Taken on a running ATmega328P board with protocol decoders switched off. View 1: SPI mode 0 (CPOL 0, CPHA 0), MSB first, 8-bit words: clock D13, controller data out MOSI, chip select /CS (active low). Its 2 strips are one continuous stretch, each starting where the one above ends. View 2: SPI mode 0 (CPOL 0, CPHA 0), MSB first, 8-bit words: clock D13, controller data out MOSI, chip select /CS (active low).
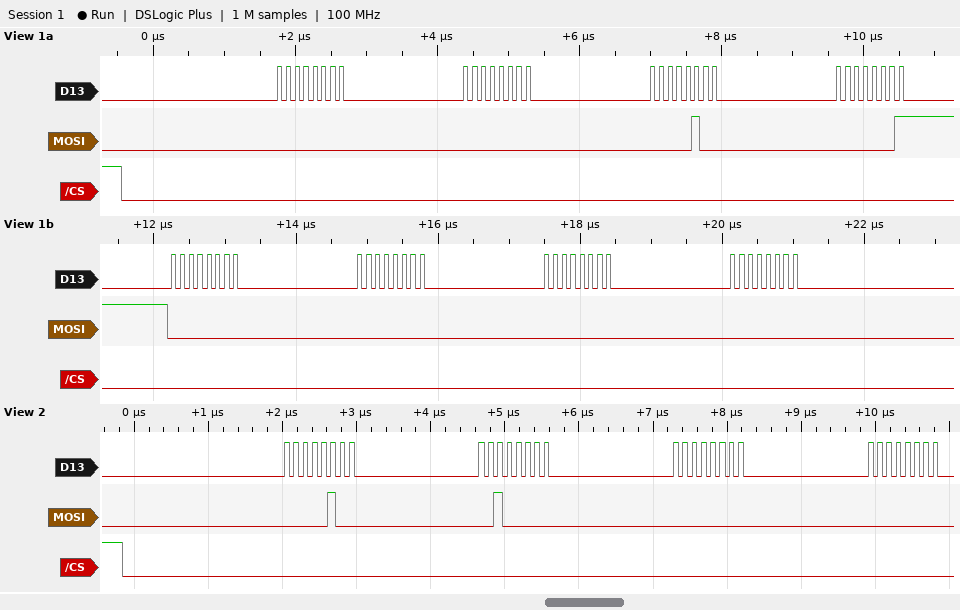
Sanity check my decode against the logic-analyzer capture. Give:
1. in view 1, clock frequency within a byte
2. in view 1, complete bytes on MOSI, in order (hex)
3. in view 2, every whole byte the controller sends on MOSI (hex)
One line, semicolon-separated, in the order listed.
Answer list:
8 MHz; 00 00 04 01 00 00 00 00; 0x04 0x20 0x00 0x00
